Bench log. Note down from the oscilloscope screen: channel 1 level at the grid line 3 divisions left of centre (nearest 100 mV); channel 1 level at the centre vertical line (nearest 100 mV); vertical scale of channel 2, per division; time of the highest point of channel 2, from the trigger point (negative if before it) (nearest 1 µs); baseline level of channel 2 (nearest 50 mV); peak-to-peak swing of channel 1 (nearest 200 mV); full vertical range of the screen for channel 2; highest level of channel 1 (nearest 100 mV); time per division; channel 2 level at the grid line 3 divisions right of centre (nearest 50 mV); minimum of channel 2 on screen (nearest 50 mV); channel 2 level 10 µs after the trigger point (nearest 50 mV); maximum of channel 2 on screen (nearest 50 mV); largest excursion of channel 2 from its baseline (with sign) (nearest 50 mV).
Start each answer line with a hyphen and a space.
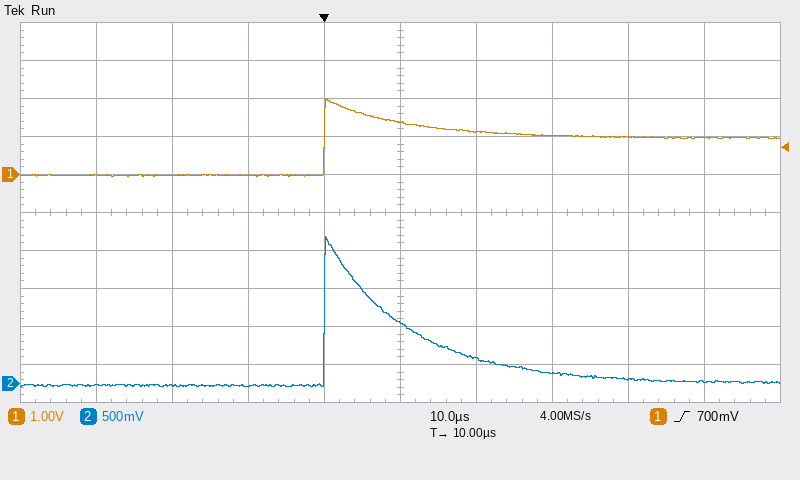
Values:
- 0.0 V
- 1.4 V
- 500 mV
- 0 µs
- 0 mV
- 2.0 V
- 5 V
- 2.0 V
- 10 µs
- 50 mV
- -50 mV
- 800 mV
- 1.95 V
- +1.95 V
